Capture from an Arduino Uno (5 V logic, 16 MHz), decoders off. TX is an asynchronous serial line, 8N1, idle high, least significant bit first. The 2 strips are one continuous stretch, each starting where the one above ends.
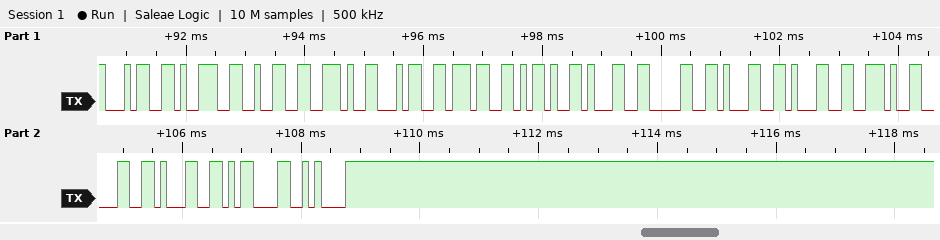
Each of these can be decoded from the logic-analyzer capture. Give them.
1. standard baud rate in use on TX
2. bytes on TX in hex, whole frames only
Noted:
9600 baud
0x34 0x39 0x32 0x2E 0x34 0x37 0x2D 0x31 0x30 0x31 0x31 0x2E 0x30 0x31 0x0D 0x0A
